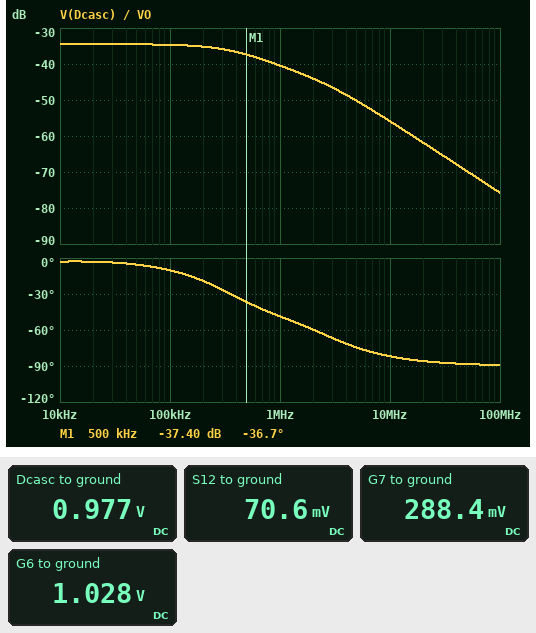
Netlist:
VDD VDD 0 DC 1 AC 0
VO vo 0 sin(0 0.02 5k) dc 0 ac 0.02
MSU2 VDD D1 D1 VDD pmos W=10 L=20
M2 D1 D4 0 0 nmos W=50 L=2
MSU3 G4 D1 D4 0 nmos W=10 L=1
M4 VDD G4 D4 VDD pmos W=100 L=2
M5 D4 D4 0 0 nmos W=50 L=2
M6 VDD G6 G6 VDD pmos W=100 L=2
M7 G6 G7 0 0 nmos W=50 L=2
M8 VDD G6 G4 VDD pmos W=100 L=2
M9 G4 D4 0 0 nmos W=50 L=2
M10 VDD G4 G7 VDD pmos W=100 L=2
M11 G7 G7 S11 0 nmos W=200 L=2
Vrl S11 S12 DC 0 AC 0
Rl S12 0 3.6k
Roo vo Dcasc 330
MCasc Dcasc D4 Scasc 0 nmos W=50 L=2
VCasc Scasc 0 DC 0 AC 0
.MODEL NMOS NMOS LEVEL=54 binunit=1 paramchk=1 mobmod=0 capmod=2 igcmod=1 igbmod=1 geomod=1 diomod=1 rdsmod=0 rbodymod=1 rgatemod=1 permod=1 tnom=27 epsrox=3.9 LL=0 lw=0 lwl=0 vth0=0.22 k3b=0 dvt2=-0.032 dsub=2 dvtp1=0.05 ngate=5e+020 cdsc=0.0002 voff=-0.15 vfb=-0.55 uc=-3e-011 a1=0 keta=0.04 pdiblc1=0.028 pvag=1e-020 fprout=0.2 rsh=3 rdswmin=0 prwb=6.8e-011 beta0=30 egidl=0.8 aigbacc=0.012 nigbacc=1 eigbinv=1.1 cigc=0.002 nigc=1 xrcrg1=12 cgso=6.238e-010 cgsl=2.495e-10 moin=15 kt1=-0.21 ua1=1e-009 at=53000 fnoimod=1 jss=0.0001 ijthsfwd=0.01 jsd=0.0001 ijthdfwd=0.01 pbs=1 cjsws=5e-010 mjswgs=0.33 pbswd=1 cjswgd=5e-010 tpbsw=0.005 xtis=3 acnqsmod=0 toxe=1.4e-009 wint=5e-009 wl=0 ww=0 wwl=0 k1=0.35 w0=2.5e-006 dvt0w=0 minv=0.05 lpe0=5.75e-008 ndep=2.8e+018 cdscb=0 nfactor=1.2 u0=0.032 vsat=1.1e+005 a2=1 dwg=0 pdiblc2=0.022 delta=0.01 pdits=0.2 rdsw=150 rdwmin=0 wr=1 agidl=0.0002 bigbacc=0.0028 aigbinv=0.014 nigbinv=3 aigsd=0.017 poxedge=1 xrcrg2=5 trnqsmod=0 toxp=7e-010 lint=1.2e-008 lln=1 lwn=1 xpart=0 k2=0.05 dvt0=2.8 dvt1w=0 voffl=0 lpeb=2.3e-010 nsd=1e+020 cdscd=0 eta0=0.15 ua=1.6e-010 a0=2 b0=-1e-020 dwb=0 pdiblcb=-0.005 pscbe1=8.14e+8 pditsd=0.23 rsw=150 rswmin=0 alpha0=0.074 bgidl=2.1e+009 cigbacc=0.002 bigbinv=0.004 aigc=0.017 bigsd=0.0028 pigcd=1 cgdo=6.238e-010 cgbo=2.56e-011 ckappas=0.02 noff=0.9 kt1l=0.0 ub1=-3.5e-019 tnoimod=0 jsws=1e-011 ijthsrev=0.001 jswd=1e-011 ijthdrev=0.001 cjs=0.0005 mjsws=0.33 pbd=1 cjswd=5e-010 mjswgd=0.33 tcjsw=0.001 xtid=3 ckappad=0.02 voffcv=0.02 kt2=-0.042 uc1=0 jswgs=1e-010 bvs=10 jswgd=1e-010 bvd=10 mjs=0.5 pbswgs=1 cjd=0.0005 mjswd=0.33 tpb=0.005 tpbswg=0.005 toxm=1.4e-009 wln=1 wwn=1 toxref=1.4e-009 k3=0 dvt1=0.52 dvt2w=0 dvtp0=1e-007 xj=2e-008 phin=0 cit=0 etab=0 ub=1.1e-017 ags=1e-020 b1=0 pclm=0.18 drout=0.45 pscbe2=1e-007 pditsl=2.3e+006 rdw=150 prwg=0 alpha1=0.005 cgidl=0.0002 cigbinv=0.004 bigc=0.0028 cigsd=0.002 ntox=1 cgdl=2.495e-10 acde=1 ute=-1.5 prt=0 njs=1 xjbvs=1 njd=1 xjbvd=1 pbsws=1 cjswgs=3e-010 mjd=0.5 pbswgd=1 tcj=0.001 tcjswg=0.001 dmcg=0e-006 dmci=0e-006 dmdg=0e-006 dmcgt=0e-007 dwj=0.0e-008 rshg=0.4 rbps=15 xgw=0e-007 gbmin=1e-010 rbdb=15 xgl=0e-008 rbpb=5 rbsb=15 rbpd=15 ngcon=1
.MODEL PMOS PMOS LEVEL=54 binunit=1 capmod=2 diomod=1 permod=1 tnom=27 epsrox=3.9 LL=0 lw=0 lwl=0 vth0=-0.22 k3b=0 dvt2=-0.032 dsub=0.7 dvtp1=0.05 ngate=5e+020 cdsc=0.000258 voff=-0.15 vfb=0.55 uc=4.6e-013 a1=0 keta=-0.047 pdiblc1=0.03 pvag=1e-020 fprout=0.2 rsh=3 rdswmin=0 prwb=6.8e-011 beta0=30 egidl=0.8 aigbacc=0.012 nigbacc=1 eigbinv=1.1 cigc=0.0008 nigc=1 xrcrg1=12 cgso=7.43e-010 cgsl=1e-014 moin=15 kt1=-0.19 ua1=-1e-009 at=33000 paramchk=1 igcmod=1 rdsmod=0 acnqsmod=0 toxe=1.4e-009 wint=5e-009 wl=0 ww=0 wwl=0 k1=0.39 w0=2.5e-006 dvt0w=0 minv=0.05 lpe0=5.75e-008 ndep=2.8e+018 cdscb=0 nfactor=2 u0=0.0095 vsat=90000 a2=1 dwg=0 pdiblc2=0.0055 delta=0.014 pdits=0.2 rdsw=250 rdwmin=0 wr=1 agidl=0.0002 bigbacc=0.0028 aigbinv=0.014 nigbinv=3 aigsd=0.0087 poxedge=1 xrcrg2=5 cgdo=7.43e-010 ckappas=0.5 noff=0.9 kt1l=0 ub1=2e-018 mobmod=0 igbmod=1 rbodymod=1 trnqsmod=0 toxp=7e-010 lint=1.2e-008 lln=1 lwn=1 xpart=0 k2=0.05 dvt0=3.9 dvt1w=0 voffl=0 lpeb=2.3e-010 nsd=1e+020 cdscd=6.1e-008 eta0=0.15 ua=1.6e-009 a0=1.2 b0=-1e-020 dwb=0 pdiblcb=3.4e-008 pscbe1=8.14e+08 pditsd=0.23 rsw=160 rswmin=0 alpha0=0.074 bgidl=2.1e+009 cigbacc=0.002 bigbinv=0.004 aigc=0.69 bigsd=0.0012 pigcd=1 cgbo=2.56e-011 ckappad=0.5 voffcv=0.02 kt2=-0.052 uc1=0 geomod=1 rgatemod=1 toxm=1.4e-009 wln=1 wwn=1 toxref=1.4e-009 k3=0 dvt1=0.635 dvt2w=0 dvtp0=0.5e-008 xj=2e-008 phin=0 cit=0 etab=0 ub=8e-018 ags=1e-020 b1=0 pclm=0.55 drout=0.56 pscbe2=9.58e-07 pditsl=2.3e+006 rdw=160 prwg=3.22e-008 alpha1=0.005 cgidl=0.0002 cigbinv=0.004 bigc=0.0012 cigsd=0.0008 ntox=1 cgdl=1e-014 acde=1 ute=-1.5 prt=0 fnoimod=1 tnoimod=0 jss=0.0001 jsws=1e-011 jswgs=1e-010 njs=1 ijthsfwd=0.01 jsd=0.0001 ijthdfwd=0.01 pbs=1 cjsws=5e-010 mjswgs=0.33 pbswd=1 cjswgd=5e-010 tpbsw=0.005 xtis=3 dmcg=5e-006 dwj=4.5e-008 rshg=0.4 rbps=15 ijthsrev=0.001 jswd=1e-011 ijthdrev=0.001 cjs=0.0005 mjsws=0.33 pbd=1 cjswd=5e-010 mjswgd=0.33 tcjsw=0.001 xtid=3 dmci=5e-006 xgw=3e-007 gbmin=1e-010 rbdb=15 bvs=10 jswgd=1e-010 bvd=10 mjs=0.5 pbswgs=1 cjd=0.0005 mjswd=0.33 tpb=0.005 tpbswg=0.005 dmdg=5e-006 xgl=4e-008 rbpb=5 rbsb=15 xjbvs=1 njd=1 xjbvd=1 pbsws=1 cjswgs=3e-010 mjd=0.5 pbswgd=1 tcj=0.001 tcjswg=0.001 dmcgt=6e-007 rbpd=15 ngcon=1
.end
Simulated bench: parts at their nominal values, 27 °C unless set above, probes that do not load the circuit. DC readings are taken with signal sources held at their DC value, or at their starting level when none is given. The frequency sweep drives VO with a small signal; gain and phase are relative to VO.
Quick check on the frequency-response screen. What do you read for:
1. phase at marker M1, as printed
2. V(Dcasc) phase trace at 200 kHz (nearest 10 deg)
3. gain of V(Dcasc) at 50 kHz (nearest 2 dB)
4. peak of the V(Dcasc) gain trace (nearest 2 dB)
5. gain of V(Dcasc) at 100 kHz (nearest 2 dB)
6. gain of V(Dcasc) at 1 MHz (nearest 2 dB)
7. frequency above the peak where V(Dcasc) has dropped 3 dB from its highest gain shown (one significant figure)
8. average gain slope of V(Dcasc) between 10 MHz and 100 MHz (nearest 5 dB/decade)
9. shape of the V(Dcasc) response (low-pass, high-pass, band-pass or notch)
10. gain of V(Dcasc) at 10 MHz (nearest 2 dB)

-36.7 deg
-20 deg
-34 dB
-34 dB
-34 dB
-40 dB
500 kHz
-20 dB/decade
low-pass
-56 dB
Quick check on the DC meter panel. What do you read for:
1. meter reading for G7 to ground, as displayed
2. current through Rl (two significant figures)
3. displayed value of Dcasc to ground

288.4 mV
20 µA
0.977 V
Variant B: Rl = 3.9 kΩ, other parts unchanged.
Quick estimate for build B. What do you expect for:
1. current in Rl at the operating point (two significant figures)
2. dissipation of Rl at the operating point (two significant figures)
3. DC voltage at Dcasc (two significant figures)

18 µA
1.3 µW
980 mV
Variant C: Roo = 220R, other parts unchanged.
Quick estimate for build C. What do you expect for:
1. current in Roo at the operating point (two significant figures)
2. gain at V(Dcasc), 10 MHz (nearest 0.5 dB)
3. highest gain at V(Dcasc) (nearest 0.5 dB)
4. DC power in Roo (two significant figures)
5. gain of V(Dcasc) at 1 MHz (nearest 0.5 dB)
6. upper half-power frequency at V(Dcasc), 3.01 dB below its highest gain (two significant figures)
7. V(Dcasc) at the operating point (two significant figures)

4.4 mA
-52.5 dB
-29.5 dB
4.2 mW
-37.0 dB
330 kHz
970 mV
